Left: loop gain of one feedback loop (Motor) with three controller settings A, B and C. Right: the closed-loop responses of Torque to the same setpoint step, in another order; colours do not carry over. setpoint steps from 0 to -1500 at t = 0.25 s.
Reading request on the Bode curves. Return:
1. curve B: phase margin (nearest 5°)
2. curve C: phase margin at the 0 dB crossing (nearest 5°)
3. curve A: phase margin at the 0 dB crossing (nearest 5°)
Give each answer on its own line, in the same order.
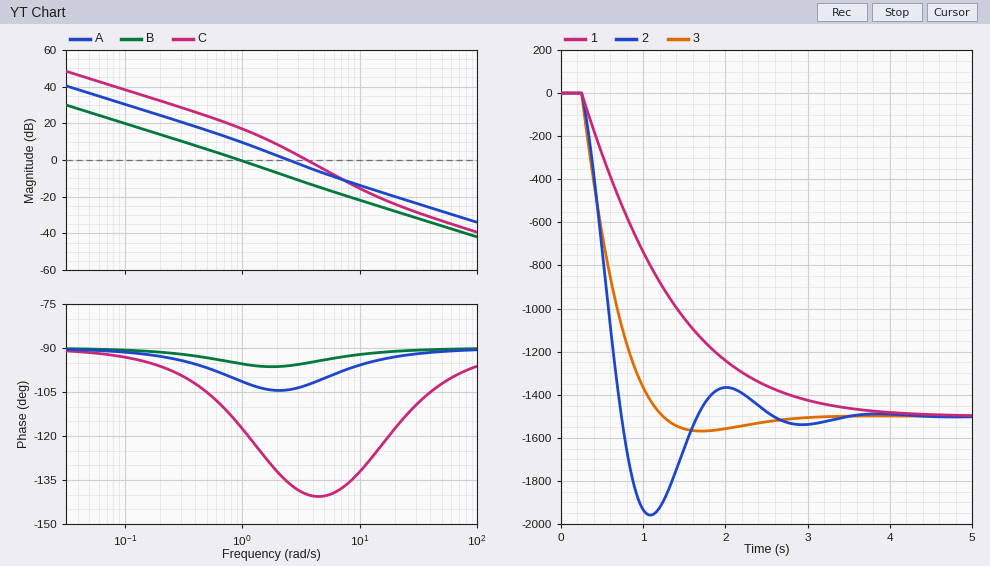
85°
40°
75°
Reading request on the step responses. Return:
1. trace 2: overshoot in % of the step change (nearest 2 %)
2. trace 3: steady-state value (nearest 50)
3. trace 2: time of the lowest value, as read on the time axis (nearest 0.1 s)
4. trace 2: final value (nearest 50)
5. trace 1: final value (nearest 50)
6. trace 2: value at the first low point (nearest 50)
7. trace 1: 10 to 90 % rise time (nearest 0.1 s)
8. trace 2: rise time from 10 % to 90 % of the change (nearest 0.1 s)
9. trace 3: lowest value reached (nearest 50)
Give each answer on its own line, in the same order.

30 %
-1500
1.1 s
-1500
-1500
-1950
2.1 s
0.4 s
-1550
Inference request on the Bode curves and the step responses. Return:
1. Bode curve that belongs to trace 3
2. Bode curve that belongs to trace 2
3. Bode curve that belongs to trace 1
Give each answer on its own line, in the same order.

A
C
B
